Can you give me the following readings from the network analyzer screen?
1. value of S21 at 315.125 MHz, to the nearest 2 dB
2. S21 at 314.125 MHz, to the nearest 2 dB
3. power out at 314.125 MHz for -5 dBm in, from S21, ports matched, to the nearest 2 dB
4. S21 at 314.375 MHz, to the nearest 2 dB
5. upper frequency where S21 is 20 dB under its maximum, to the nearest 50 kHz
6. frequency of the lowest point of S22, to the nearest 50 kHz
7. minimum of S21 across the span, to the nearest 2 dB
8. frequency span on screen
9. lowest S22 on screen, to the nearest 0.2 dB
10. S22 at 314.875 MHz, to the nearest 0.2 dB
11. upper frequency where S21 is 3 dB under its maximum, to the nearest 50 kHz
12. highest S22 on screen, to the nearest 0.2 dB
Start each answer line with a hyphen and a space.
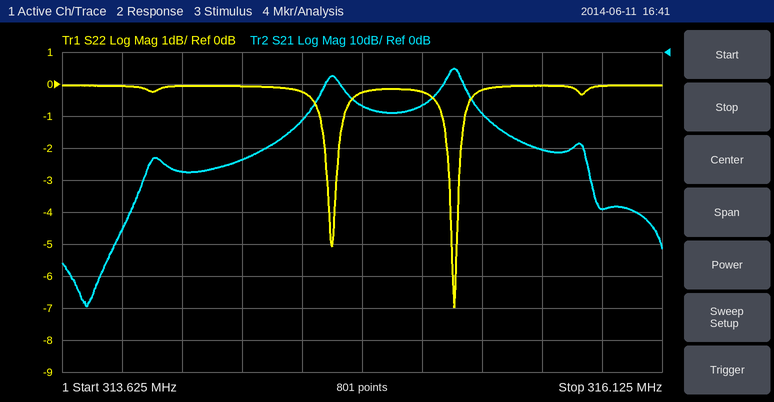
- -16 dB
- -38 dB
- -42 dBm
- -34 dB
- 315.45 MHz
- 315.25 MHz
- -80 dB
- 2.5 MHz
- -7.0 dB
- -0.2 dB
- 315.30 MHz
- 0.0 dB
